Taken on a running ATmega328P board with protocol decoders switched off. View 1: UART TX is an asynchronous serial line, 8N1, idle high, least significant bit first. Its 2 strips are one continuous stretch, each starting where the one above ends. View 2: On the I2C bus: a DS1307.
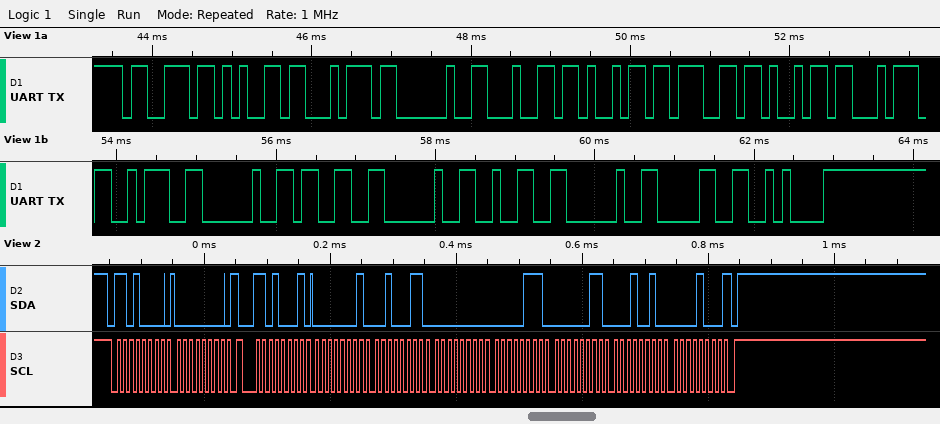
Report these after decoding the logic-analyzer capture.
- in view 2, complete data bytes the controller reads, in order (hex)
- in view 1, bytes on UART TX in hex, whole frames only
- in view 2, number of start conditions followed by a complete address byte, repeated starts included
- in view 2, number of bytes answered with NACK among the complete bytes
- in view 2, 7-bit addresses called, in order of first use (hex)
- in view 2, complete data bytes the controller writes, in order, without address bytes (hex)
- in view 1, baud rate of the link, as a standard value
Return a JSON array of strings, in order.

["01 23 00 07 03 12 08", "0x73 0x65 0x74 0x20 0x64 0x69 0x67 0x69 0x74 0x3A 0x20 0x33 0x20 0x32 0x20 0x30 0x0A", "2", "1", "0x68", "00", "9600 baud"]
